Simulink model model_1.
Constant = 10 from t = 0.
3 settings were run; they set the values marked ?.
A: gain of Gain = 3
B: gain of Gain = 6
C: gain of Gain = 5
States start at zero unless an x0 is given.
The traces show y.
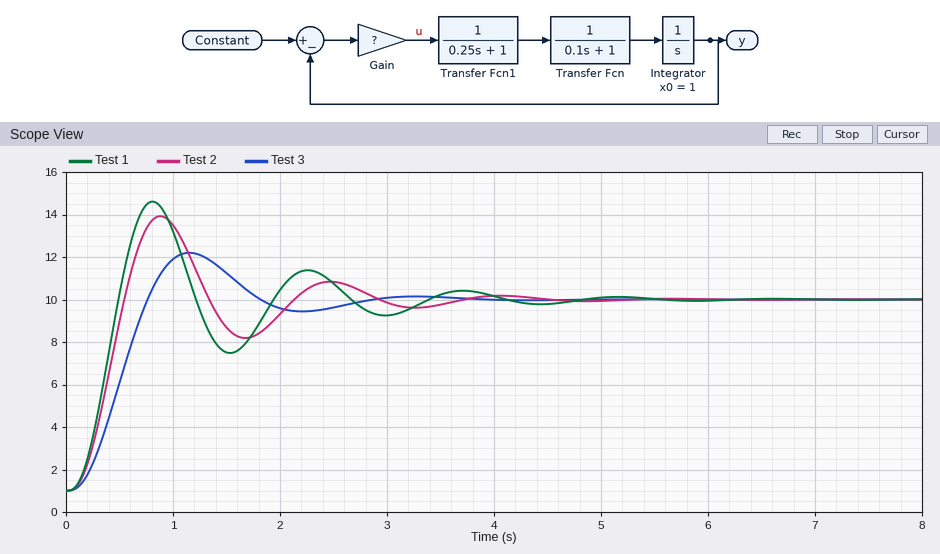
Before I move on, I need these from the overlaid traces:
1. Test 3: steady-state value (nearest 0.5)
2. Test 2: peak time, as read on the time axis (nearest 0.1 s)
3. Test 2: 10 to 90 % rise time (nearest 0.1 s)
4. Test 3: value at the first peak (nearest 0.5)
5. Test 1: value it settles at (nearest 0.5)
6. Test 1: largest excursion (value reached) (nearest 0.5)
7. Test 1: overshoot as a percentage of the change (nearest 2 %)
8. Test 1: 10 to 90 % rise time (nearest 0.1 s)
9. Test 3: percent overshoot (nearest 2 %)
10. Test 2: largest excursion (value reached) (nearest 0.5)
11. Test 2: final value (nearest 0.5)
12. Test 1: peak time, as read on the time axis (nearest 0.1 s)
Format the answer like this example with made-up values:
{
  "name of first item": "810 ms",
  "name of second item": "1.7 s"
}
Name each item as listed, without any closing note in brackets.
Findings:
{
  "Test 3: steady-state value": "10.0",
  "Test 2: peak time, as read on the time axis": "0.9 s",
  "Test 2: 10 to 90 % rise time": "0.3 s",
  "Test 3: value at the first peak": "12.0",
  "Test 1: value it settles at": "10.0",
  "Test 1: largest excursion (value reached)": "14.5",
  "Test 1: overshoot as a percentage of the change": "52 %",
  "Test 1: 10 to 90 % rise time": "0.3 s",
  "Test 3: percent overshoot": "24 %",
  "Test 2: largest excursion (value reached)": "14.0",
  "Test 2: final value": "10.0",
  "Test 1: peak time, as read on the time axis": "0.8 s"
}
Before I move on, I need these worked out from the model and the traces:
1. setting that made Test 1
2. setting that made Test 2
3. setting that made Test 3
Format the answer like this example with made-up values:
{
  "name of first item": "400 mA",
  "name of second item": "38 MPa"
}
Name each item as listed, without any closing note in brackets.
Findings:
{
  "setting that made Test 1": "B",
  "setting that made Test 2": "C",
  "setting that made Test 3": "A"
}
